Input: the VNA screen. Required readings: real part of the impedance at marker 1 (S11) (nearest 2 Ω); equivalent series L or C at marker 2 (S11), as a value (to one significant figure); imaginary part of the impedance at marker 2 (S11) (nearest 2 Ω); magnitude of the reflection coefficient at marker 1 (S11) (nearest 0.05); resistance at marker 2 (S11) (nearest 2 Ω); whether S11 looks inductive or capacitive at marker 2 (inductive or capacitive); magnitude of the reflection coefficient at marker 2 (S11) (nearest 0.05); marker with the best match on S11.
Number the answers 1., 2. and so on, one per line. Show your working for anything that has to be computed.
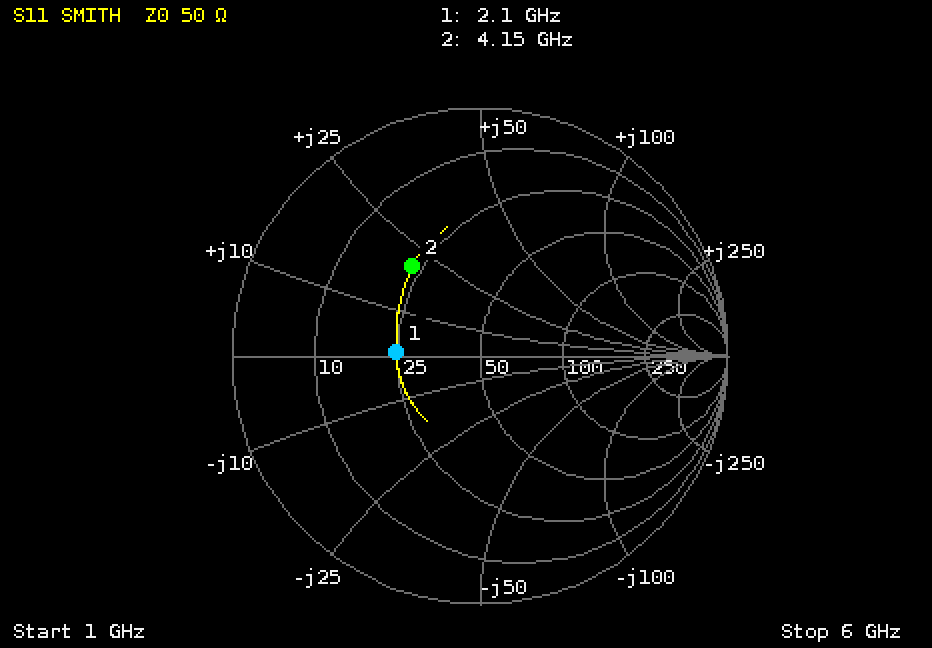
1. 24 Ω
2. L = 20 Ω/(2π × 4.15 GHz) ≈ 767 pH, so 800 pH to one significant figure
3. +20 Ω
4. 0.35
5. 22 Ω
6. inductive
7. 0.45
8. marker 1
